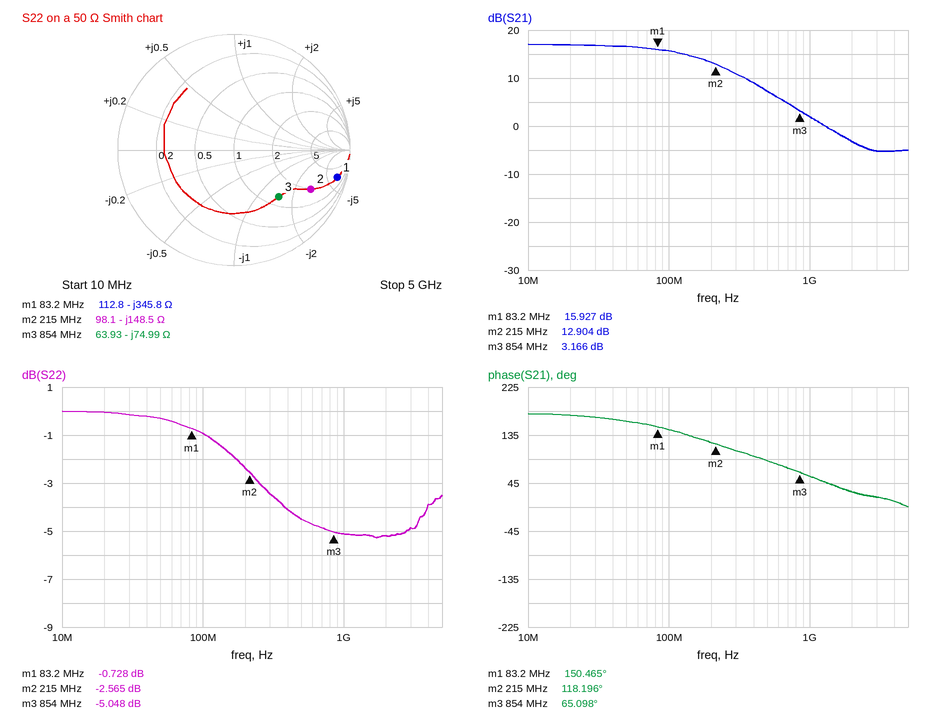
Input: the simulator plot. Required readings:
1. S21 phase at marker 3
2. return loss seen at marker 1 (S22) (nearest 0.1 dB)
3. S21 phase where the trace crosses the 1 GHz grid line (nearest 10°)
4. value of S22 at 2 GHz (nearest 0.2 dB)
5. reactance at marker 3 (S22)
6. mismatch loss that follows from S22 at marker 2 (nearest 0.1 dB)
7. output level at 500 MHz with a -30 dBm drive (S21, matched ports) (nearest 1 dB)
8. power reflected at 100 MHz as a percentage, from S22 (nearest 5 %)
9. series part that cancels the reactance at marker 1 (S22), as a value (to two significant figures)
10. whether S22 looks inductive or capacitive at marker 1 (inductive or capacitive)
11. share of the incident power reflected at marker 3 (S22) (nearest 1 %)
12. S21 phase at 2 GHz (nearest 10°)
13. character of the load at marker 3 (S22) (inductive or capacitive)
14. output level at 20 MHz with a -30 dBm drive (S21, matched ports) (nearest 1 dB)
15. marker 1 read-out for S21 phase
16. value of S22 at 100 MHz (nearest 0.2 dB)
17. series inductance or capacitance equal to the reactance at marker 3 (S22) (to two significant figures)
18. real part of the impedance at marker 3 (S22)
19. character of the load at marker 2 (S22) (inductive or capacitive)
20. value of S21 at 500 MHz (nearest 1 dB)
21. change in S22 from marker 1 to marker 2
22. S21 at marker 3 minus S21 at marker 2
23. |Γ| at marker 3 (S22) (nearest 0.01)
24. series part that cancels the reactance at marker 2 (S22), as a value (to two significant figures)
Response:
65.098°
0.7 dB
60°
-5.2 dB
-74.99 Ω
3.5 dB
-23 dBm
80 %
660 nH
capacitive
31 %
30°
capacitive
-13 dBm
150.465°
-1.0 dB
2.5 pF
63.93 Ω
capacitive
7 dB
-1.837 dB
-9.738 dB
0.56
110 nH
